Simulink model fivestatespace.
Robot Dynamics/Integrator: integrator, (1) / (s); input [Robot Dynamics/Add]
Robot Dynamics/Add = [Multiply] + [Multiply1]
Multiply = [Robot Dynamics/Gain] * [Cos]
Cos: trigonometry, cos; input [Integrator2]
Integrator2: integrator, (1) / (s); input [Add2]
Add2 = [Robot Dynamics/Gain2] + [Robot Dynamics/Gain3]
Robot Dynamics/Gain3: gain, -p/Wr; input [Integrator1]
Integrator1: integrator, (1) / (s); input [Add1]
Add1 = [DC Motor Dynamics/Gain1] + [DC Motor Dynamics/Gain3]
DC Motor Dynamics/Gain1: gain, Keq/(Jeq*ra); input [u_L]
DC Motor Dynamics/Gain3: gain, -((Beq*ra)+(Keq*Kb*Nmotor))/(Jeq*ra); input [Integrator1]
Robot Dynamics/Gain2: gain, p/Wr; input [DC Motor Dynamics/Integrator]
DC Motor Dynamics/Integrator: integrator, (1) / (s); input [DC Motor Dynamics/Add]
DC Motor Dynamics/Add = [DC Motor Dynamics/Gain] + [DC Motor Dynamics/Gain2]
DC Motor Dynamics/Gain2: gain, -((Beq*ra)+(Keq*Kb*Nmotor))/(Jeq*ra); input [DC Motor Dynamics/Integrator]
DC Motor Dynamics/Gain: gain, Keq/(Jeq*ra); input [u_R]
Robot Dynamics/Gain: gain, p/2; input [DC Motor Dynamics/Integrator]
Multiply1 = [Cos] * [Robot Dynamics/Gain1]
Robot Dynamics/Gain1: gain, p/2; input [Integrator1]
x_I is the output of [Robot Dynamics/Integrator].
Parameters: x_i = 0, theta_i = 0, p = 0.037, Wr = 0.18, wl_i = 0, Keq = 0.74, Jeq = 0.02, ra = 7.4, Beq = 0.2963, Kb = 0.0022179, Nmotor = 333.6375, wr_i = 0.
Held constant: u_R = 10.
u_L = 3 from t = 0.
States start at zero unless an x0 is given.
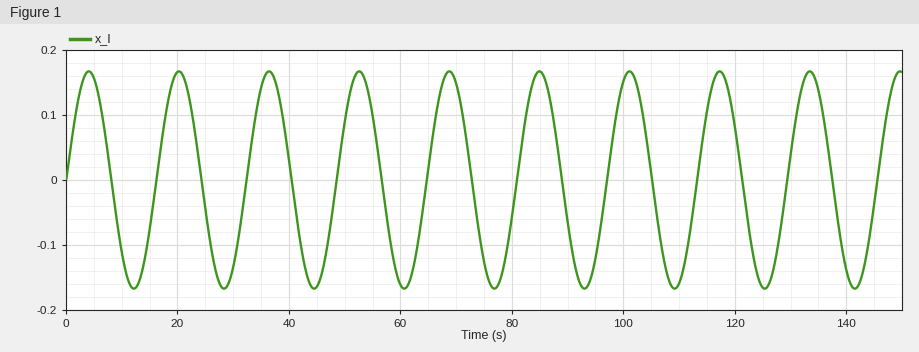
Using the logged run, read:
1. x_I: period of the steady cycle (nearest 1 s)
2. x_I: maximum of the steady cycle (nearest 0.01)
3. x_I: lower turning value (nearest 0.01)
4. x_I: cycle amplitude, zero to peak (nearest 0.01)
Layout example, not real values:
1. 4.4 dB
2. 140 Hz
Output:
1. 16 s
2. 0.17
3. -0.17
4. 0.17
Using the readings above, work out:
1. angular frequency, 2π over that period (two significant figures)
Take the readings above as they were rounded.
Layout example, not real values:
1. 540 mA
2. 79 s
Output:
1. 0.39 rad/s
